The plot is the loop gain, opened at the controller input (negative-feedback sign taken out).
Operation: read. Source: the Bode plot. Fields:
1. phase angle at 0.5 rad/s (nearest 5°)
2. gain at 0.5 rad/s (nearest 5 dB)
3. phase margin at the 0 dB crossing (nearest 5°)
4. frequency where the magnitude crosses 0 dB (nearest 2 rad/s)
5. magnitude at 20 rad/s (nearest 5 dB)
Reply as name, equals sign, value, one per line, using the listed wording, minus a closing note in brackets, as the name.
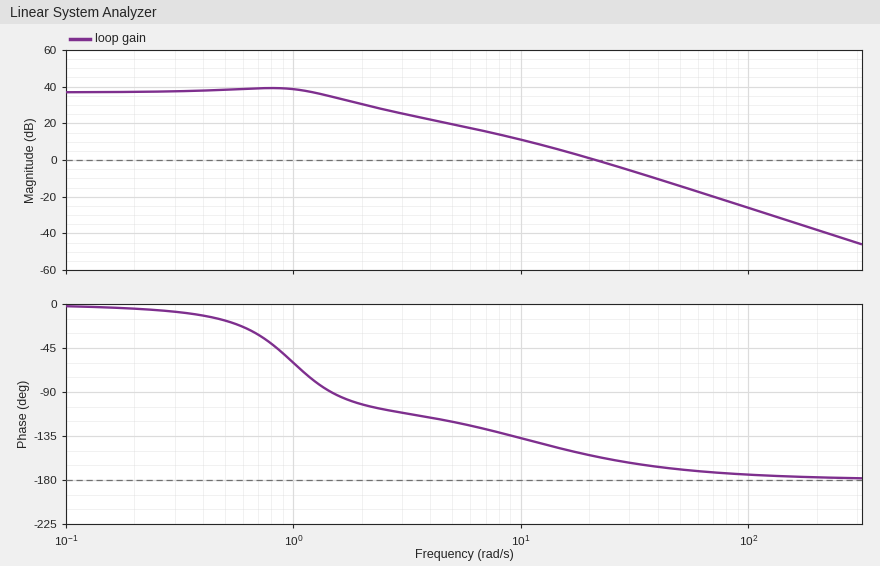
phase angle at 0.5 rad/s = -15°
gain at 0.5 rad/s = 40 dB
phase margin at the 0 dB crossing = 25°
frequency where the magnitude crosses 0 dB = 22 rad/s
magnitude at 20 rad/s = 0 dB
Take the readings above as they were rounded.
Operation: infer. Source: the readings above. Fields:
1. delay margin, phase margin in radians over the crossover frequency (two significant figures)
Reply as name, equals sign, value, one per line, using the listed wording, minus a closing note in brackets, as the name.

delay margin, phase margin in radians over the crossover frequency = 0.020 s
